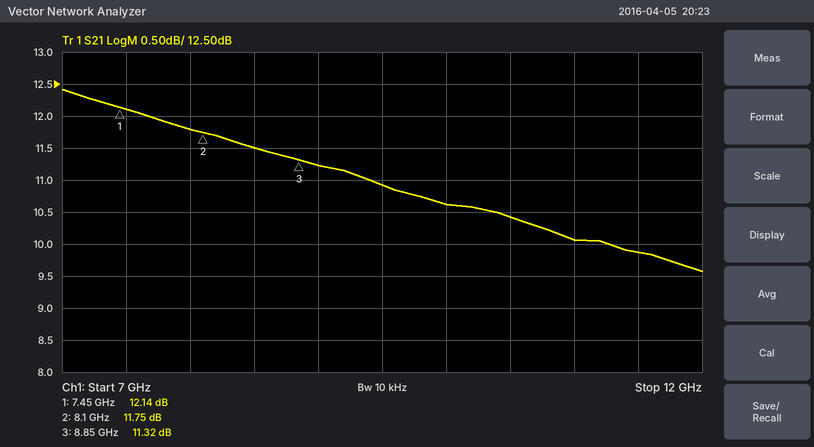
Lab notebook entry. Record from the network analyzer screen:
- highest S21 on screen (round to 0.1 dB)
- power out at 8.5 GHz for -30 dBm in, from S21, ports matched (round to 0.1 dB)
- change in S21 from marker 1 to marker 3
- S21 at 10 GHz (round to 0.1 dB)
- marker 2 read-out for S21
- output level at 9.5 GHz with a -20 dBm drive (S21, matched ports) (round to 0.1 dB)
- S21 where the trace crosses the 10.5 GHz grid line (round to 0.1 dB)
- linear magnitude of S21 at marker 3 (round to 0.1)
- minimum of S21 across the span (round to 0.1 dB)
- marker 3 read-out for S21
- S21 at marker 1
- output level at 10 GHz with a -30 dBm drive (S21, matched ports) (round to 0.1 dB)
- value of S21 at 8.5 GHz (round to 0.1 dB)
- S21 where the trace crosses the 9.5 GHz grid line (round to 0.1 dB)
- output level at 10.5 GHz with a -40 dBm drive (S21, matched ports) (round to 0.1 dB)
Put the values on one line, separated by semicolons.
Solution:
12.4 dB; -18.5 dBm; -0.82 dB; 10.6 dB; 11.75 dB; -9.1 dBm; 10.4 dB; 3.7; 9.6 dB; 11.32 dB; 12.14 dB; -19.4 dBm; 11.5 dB; 10.9 dB; -29.6 dBm
